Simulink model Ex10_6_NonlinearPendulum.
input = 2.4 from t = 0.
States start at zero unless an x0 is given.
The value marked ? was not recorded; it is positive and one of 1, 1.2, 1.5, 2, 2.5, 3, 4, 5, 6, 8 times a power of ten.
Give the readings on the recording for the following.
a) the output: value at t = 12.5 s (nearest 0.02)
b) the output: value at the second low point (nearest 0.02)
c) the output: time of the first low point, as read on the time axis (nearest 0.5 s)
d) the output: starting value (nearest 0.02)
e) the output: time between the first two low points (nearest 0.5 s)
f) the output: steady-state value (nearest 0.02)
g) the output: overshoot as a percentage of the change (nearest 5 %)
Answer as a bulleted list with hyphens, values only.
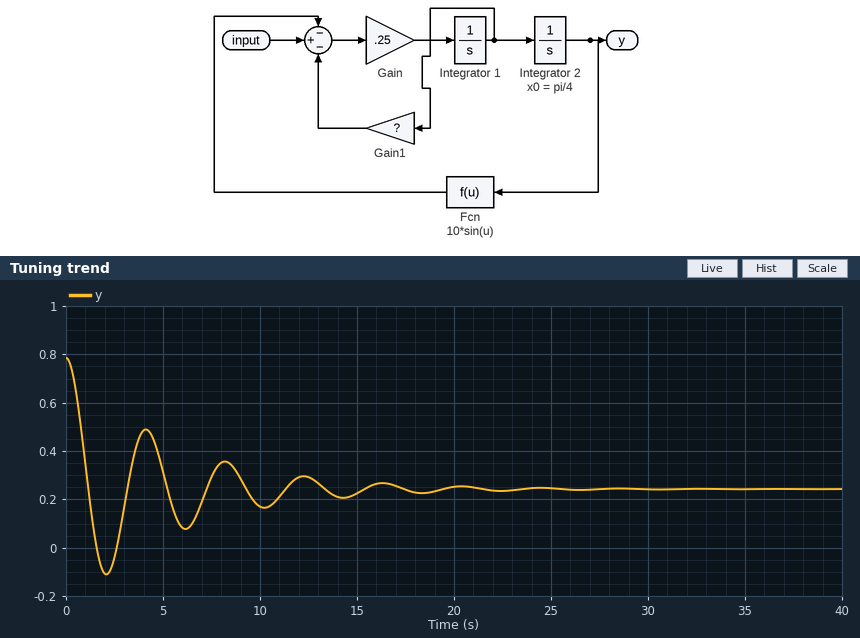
- 0.30
- 0.08
- 2.0 s
- 0.78
- 4.0 s
- 0.24
- 65 %
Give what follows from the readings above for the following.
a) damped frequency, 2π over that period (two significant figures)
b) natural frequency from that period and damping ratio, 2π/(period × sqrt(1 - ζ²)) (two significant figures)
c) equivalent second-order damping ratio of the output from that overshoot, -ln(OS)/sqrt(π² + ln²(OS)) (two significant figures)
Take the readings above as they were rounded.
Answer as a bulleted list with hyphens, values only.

- 1.6 rad/s
- 1.6 rad/s
- 0.14
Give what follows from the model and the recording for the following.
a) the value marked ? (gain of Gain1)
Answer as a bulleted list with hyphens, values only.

- 1.5
